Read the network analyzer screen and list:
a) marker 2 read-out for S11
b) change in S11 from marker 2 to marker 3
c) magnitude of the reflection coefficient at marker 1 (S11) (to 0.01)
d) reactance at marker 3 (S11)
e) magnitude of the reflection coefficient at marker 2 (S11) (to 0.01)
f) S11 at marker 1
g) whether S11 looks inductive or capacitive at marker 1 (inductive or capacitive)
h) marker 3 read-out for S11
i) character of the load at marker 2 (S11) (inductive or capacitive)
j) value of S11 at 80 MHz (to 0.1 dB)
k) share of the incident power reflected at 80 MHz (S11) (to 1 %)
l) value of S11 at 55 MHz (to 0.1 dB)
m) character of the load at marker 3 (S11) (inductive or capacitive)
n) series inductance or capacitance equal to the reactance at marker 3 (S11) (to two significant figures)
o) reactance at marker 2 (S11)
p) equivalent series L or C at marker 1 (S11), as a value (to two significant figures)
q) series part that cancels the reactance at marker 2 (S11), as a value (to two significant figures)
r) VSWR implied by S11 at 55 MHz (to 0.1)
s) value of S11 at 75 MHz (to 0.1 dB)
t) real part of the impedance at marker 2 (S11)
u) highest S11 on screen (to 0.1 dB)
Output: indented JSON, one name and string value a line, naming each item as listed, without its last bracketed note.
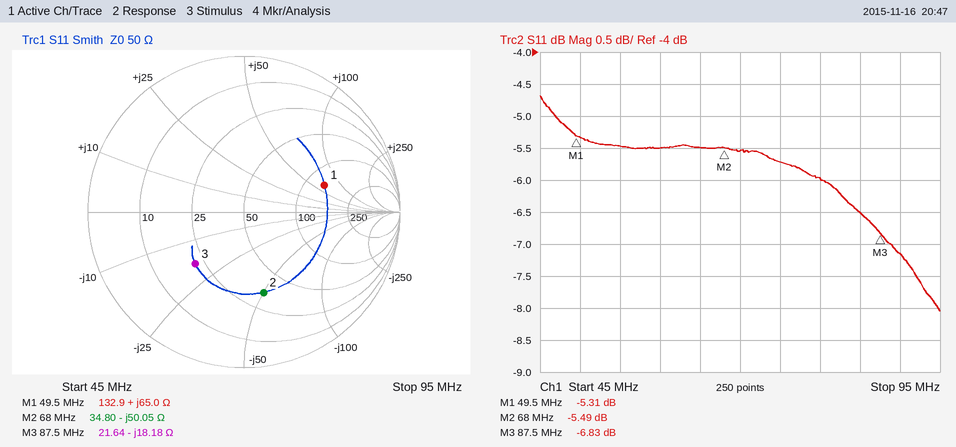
{
  "marker 2 read-out for S11": "-5.49 dB",
  "change in S11 from marker 2 to marker 3": "-1.34 dB",
  "magnitude of the reflection coefficient at marker 1 (S11)": "0.54",
  "reactance at marker 3": "-18.18 Ω",
  "magnitude of the reflection coefficient at marker 2 (S11)": "0.53",
  "S11 at marker 1": "-5.31 dB",
  "whether S11 looks inductive or capacitive at marker 1": "inductive",
  "marker 3 read-out for S11": "-6.83 dB",
  "character of the load at marker 2 (S11)": "capacitive",
  "value of S11 at 80 MHz": "-6.0 dB",
  "share of the incident power reflected at 80 MHz (S11)": "25 %",
  "value of S11 at 55 MHz": "-5.5 dB",
  "character of the load at marker 3 (S11)": "capacitive",
  "series inductance or capacitance equal to the reactance at marker 3 (S11)": "100 pF",
  "reactance at marker 2": "-50.05 Ω",
  "equivalent series L or C at marker 1 (S11), as a value": "210 nH",
  "series part that cancels the reactance at marker 2 (S11), as a value": "120 nH",
  "VSWR implied by S11 at 55 MHz": "3.3",
  "value of S11 at 75 MHz": "-5.7 dB",
  "real part of the impedance at marker 2": "34.80 Ω",
  "highest S11 on screen": "-4.7 dB"
}
